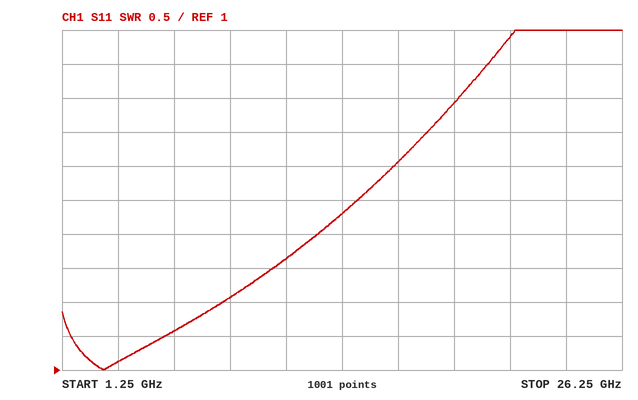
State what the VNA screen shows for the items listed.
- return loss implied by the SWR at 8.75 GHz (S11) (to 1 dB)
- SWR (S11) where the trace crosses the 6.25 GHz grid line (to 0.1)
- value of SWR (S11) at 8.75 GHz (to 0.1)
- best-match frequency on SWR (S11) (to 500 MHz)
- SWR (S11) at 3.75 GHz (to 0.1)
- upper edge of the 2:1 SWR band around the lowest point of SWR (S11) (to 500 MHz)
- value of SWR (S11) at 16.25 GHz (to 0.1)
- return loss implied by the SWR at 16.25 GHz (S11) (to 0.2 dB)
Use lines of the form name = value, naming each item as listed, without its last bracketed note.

return loss implied by the SWR at 8.75 GHz (S11) = 9 dB
SWR (S11) where the trace crosses the 6.25 GHz grid line = 1.6
value of SWR (S11) at 8.75 GHz = 2.1
best-match frequency on SWR (S11) = 3.0 GHz
SWR (S11) at 3.75 GHz = 1.1
upper edge of the 2:1 SWR band around the lowest point of SWR (S11) = 8.5 GHz
value of SWR (S11) at 16.25 GHz = 4.1
return loss implied by the SWR at 16.25 GHz (S11) = 4.4 dB
